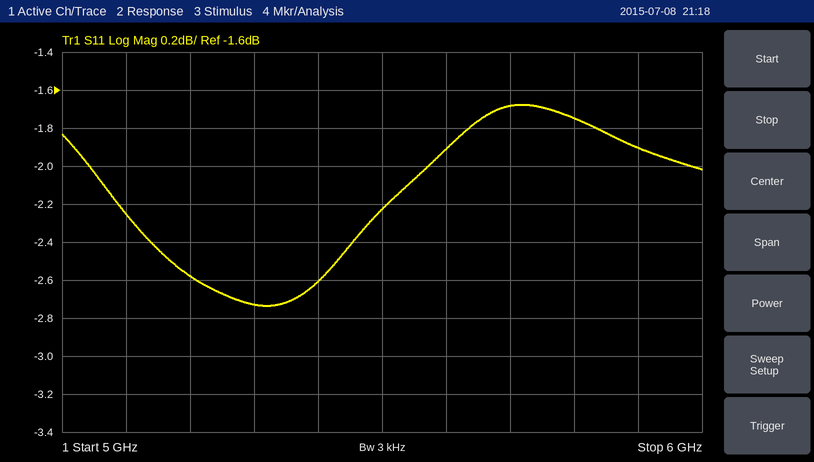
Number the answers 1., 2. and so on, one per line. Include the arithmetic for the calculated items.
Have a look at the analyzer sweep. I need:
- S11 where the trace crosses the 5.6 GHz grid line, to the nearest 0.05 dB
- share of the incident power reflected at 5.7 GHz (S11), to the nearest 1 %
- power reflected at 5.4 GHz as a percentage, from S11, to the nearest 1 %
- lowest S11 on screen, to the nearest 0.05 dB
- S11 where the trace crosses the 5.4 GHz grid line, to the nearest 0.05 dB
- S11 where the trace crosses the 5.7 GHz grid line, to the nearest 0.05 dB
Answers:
1. -1.90 dB
2. 10^(-1.7/10) ≈ 68 %
3. 10^(-2.6/10) ≈ 55 %
4. -2.75 dB
5. -2.60 dB
6. -1.70 dB
